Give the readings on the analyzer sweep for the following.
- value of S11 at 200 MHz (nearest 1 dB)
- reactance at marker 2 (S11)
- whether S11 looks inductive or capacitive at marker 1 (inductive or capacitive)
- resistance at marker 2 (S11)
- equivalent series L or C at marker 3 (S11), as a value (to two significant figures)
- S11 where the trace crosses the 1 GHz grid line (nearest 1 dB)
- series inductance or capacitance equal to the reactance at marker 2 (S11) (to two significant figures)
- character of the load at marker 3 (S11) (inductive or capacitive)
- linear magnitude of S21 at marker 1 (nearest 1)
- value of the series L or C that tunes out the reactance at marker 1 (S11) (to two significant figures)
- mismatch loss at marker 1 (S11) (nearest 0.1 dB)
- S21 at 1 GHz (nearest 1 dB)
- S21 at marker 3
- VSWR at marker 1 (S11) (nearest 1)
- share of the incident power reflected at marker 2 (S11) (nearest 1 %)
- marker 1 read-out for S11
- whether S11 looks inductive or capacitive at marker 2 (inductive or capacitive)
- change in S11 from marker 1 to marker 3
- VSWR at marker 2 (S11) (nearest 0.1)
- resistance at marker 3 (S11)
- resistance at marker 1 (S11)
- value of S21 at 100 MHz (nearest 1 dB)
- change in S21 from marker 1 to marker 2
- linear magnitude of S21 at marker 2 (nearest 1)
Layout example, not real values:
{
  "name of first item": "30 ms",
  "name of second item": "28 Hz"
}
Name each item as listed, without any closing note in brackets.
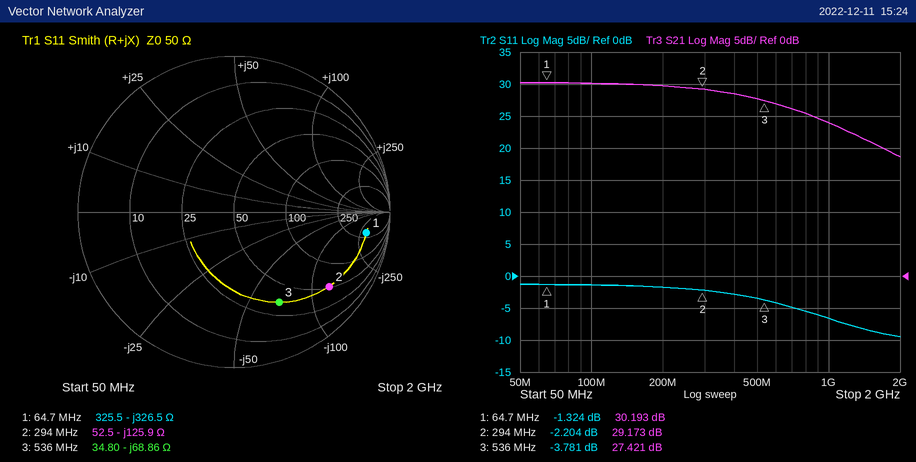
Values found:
{
  "value of S11 at 200 MHz": "-2 dB",
  "reactance at marker 2": "-125.9 Ω",
  "whether S11 looks inductive or capacitive at marker 1": "capacitive",
  "resistance at marker 2": "52.5 Ω",
  "equivalent series L or C at marker 3 (S11), as a value": "4.3 pF",
  "S11 where the trace crosses the 1 GHz grid line": "-7 dB",
  "series inductance or capacitance equal to the reactance at marker 2 (S11)": "4.3 pF",
  "character of the load at marker 3 (S11)": "capacitive",
  "linear magnitude of S21 at marker 1": "32",
  "value of the series L or C that tunes out the reactance at marker 1 (S11)": "800 nH",
  "mismatch loss at marker 1 (S11)": "5.8 dB",
  "S21 at 1 GHz": "24 dB",
  "S21 at marker 3": "27.421 dB",
  "VSWR at marker 1 (S11)": "13",
  "share of the incident power reflected at marker 2 (S11)": "60 %",
  "marker 1 read-out for S11": "-1.324 dB",
  "whether S11 looks inductive or capacitive at marker 2": "capacitive",
  "change in S11 from marker 1 to marker 3": "-2.457 dB",
  "VSWR at marker 2 (S11)": "7.9",
  "resistance at marker 3": "34.80 Ω",
  "resistance at marker 1": "325.5 Ω",
  "value of S21 at 100 MHz": "30 dB",
  "change in S21 from marker 1 to marker 2": "-1.020 dB",
  "linear magnitude of S21 at marker 2": "29"
}
